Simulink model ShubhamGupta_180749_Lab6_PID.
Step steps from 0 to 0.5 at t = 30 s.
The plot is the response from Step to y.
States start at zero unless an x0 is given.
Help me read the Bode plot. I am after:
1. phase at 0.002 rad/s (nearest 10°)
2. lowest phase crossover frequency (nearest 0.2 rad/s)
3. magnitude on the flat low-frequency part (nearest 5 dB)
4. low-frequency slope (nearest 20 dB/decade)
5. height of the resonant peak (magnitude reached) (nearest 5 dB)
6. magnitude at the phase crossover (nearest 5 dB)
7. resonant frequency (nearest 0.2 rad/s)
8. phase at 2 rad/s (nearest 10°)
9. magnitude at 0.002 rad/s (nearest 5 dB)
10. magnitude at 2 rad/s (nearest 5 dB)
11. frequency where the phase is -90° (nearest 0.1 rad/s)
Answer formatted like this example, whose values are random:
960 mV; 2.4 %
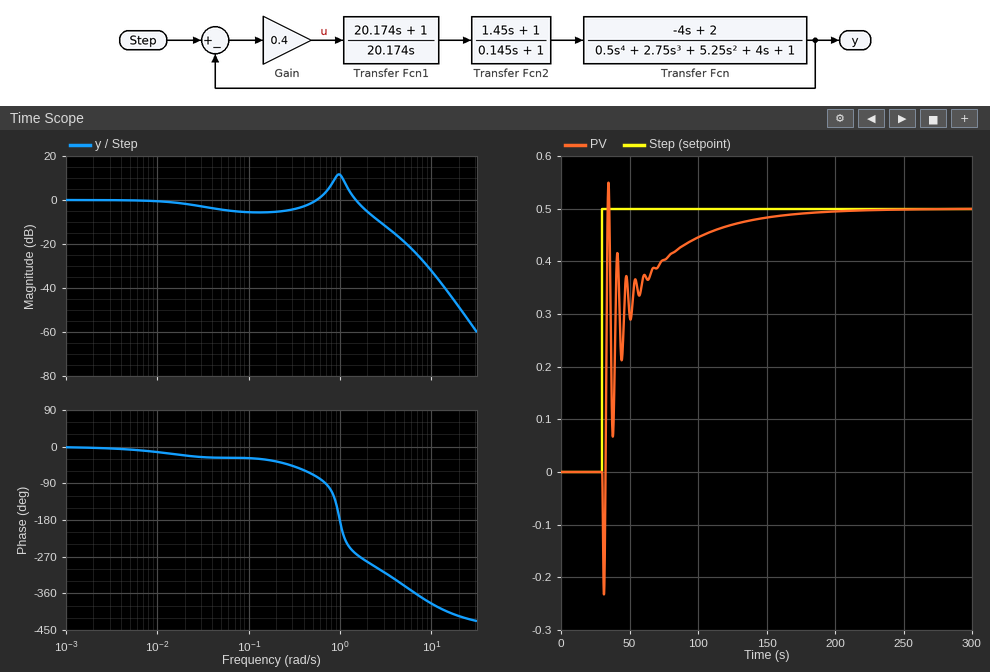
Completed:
0°; 1.0 rad/s; 0 dB; 0 dB/decade; 10 dB; 10 dB; 1.0 rad/s; -280°; 0 dB; -5 dB; 0.7 rad/s
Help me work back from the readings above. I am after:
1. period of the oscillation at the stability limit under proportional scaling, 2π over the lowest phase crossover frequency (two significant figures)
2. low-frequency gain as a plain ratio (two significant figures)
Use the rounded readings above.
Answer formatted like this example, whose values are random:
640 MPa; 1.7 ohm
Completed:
6.3 s; 1.0
